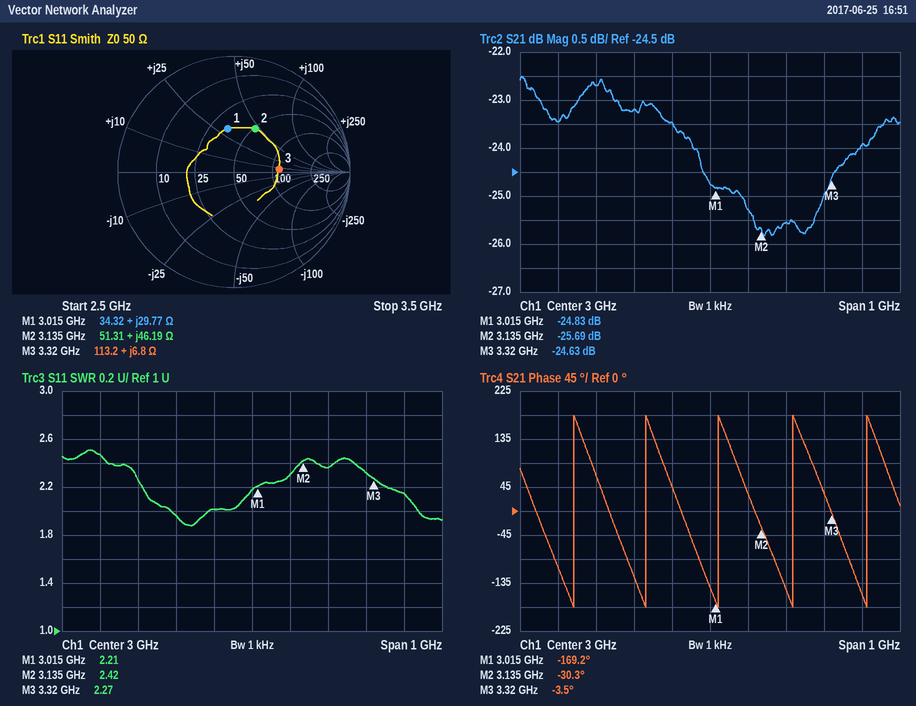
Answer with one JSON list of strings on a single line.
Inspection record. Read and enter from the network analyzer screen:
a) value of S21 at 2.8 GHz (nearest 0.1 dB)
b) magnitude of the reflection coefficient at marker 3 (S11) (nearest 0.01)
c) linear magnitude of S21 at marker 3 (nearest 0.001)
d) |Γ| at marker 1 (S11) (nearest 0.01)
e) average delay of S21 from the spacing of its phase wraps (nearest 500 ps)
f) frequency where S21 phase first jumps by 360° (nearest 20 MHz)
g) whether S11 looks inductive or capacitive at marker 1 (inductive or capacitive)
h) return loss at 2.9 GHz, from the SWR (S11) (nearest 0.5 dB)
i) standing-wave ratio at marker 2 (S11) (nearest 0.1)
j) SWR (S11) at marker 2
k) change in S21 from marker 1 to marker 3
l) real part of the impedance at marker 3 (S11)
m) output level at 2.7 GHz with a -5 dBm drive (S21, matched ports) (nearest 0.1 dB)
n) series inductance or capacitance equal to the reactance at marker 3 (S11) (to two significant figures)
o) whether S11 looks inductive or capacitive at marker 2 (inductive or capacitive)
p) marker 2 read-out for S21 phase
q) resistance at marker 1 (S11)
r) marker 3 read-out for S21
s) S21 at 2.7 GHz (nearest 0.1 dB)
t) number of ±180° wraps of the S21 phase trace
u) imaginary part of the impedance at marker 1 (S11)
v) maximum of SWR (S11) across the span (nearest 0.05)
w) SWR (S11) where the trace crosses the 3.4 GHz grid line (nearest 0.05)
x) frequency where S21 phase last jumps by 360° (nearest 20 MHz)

["-23.2 dB", "0.39", "0.059", "0.38", "5.0 ns", "2.64 GHz", "inductive", "9.5 dB", "2.4", "2.42", "0.20 dB", "113.2 Ω", "-27.7 dBm", "330 pH", "inductive", "-30.3°", "34.32 Ω", "-24.63 dB", "-22.7 dB", "5", "+29.77 Ω", "2.50", "2.15", "3.42 GHz"]
